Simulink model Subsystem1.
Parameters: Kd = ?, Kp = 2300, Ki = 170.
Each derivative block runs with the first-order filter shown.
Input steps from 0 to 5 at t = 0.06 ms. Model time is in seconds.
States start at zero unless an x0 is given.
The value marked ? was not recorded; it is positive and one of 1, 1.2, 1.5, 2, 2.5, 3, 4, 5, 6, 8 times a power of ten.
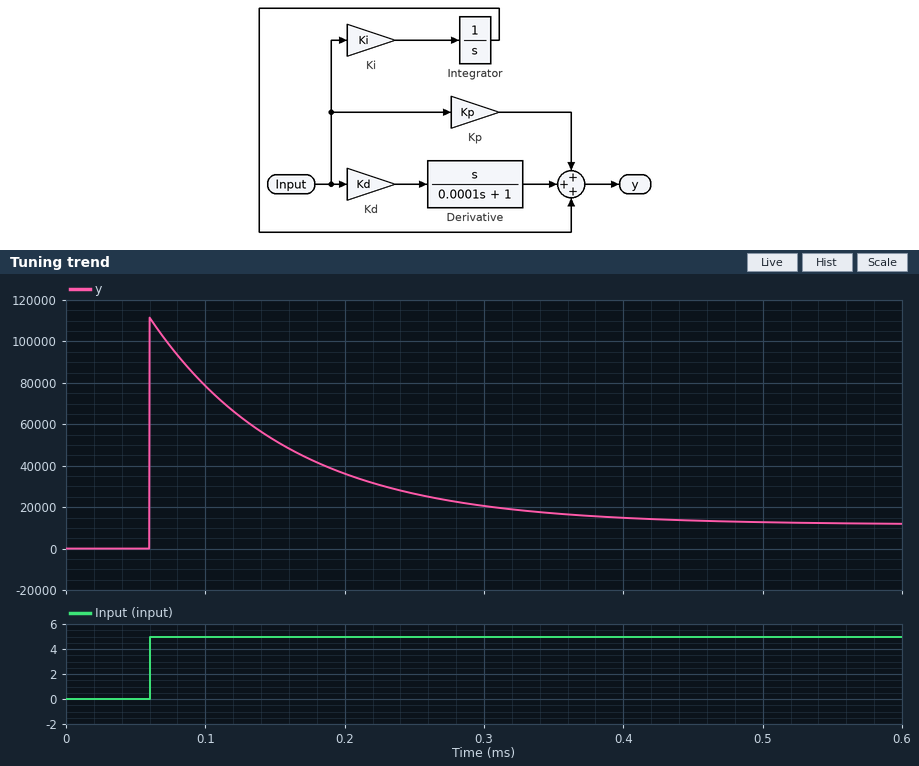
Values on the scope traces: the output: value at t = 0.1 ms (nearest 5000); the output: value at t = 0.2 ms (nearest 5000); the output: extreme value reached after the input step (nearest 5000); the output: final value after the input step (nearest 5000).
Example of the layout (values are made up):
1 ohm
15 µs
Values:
80000
35000
110000
10000
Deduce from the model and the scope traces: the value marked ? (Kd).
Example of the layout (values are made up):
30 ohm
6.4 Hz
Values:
2
